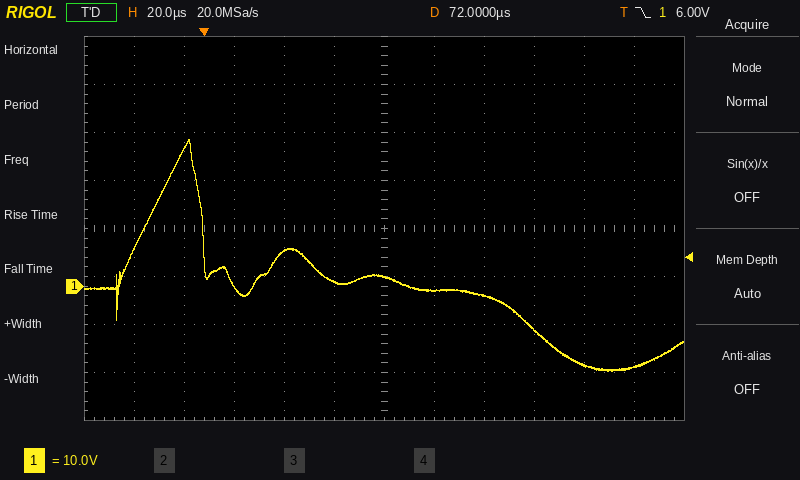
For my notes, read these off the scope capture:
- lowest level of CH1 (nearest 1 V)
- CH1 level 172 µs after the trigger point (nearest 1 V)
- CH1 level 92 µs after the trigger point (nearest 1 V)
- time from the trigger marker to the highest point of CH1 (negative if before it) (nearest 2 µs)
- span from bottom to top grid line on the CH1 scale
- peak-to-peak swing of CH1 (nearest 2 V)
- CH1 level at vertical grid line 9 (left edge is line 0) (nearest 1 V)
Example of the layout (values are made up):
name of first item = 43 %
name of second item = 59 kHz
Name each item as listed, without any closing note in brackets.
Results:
lowest level of CH1 = -18 V
CH1 level 172 µs after the trigger point = -17 V
CH1 level 92 µs after the trigger point = -1 V
time from the trigger marker to the highest point of CH1 (negative if before it) = -6 µs
span from bottom to top grid line on the CH1 scale = 80 V
peak-to-peak swing of CH1 = 48 V
CH1 level at vertical grid line 9 (left edge is line 0) = -9 V
